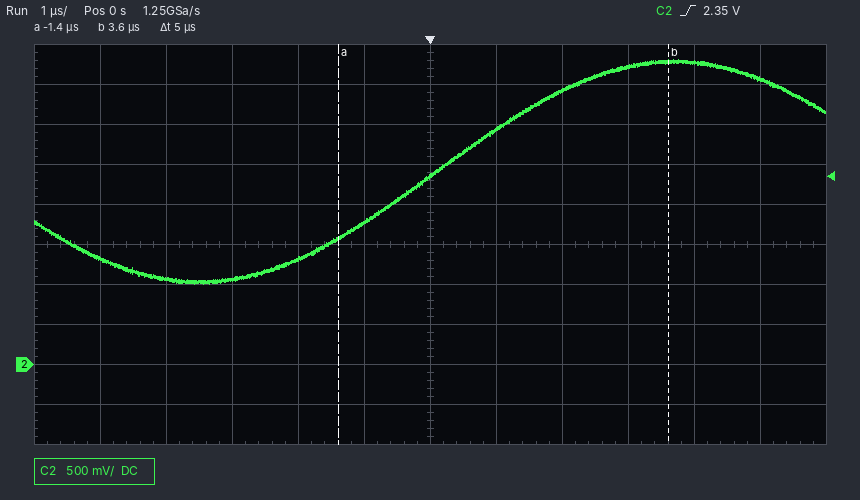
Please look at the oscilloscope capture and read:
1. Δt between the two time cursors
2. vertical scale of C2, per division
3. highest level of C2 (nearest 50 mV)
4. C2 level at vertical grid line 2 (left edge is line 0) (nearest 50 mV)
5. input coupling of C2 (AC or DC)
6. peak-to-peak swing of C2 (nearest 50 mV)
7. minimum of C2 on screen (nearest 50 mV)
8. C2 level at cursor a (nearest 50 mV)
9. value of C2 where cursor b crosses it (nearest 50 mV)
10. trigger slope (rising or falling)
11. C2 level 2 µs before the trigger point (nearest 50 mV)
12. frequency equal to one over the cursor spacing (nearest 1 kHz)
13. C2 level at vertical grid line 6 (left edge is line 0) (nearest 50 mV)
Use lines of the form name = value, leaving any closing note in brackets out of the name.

Δt between the two time cursors = 5 µs
vertical scale of C2, per division = 500 mV
highest level of C2 = 3.80 V
C2 level at vertical grid line 2 (left edge is line 0) = 1.05 V
input coupling of C2 = DC
peak-to-peak swing of C2 = 2.80 V
minimum of C2 on screen = 1.00 V
C2 level at cursor a = 1.55 V
value of C2 where cursor b crosses it = 3.80 V
trigger slope = rising
C2 level 2 µs before the trigger point = 1.30 V
frequency equal to one over the cursor spacing = 200 kHz
C2 level at vertical grid line 6 (left edge is line 0) = 2.35 V
